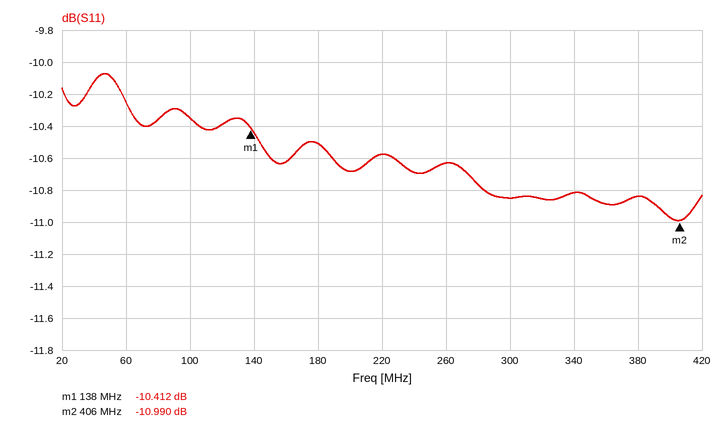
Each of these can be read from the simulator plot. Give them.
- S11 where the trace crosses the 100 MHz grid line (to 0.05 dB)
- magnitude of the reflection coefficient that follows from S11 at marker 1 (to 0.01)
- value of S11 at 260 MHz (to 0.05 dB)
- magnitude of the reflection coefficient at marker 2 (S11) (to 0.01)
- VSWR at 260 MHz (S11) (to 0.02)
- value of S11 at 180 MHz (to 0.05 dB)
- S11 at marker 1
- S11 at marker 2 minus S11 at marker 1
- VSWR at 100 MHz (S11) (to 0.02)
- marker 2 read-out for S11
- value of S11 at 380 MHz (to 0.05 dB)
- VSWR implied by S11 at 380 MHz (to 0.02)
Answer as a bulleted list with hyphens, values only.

- -10.35 dB
- 0.30
- -10.65 dB
- 0.28
- 1.84
- -10.50 dB
- -10.412 dB
- -0.578 dB
- 1.88
- -10.990 dB
- -10.85 dB
- 1.80
